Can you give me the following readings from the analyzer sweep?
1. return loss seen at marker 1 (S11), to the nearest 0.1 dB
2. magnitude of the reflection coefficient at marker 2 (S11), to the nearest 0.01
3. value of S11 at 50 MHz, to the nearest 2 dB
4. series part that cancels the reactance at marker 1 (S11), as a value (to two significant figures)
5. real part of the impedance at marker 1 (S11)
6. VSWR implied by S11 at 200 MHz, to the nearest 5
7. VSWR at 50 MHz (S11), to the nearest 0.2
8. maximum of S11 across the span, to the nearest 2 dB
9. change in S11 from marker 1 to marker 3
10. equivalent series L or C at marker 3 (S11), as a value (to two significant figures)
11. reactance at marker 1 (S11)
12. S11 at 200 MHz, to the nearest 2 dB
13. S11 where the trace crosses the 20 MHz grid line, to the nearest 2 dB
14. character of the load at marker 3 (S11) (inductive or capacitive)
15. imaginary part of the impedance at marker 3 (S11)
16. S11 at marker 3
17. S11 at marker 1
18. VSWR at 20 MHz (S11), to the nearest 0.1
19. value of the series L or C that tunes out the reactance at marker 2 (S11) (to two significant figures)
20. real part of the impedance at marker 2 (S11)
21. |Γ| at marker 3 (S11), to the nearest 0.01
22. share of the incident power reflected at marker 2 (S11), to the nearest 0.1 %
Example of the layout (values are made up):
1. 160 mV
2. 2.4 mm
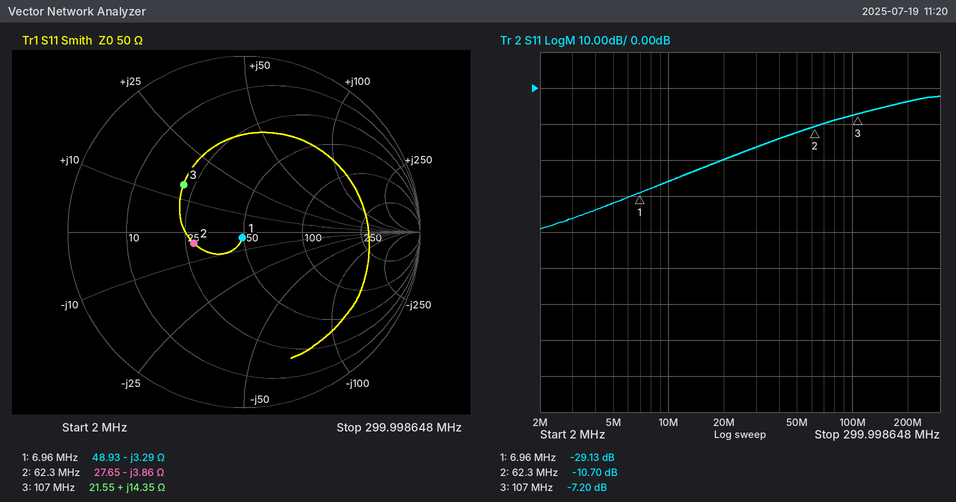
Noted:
1. 29.1 dB
2. 0.29
3. -12 dB
4. 75 nH
5. 48.93 Ω
6. 5
7. 1.6
8. -2 dB
9. 21.93 dB
10. 21 nH
11. -3.29 Ω
12. -4 dB
13. -20 dB
14. inductive
15. +14.35 Ω
16. -7.20 dB
17. -29.13 dB
18. 1.2
19. 9.9 nH
20. 27.65 Ω
21. 0.44
22. 8.5 %
